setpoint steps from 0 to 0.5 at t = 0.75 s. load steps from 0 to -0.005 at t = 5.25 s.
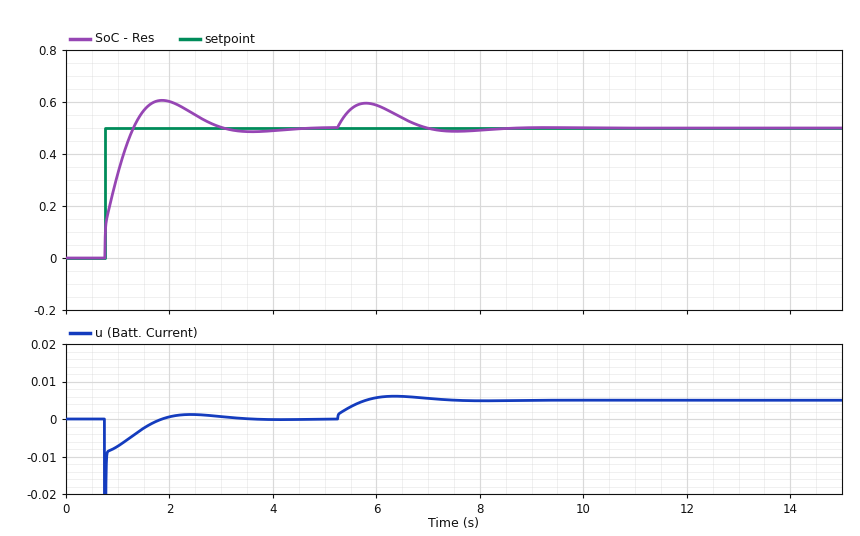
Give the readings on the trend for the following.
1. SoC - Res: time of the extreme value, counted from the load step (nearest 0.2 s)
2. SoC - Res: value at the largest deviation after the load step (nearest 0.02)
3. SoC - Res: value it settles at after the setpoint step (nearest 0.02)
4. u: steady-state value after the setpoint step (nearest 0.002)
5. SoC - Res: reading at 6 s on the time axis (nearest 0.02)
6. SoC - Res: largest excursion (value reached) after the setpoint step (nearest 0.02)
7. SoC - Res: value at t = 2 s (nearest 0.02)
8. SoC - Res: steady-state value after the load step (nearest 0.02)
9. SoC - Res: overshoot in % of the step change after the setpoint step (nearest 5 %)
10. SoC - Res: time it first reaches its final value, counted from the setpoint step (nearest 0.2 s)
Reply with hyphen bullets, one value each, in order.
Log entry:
- 0.6 s
- 0.60
- 0.50
- 0.000
- 0.58
- 0.60
- 0.60
- 0.50
- 20 %
- 0.6 s
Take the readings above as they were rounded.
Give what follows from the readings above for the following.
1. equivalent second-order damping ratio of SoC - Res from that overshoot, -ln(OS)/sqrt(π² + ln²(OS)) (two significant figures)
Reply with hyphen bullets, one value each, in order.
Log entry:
- 0.46
